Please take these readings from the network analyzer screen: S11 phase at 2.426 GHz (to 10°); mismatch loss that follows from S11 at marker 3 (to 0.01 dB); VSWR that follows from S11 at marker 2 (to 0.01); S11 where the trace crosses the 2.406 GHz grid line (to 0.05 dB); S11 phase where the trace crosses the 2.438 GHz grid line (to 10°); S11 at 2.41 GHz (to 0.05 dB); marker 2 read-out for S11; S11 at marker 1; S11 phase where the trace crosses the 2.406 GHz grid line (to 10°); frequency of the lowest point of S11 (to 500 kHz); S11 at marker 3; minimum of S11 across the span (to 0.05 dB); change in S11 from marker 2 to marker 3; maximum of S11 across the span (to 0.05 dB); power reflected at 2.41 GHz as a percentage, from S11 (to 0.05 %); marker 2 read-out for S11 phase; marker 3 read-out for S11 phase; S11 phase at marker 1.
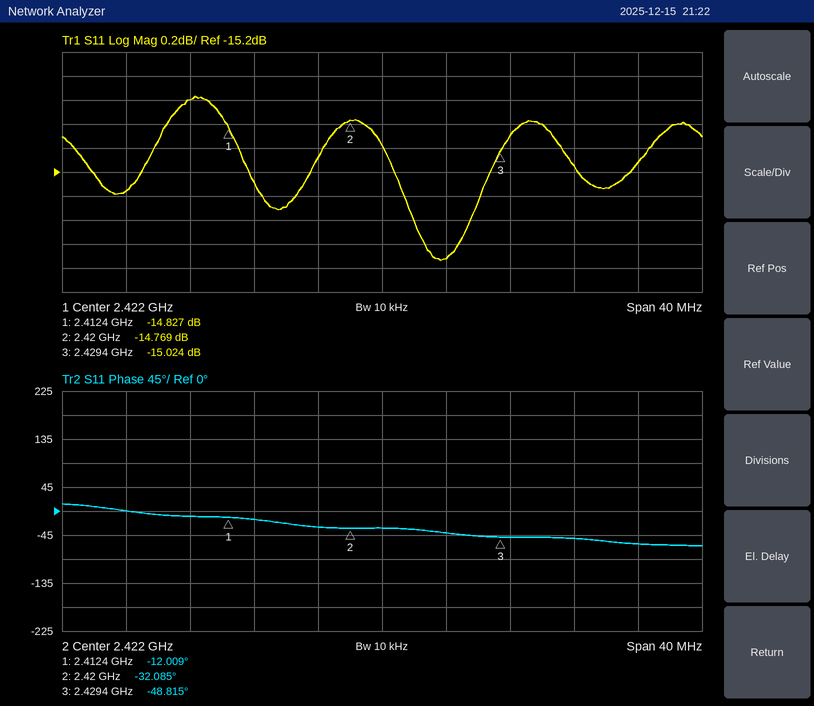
-40°
0.14 dB
1.45
-15.35 dB
-60°
-14.60 dB
-14.769 dB
-14.827 dB
0°
2.4255 GHz
-15.024 dB
-15.95 dB
-0.255 dB
-14.55 dB
3.45 %
-32.085°
-48.815°
-12.009°
